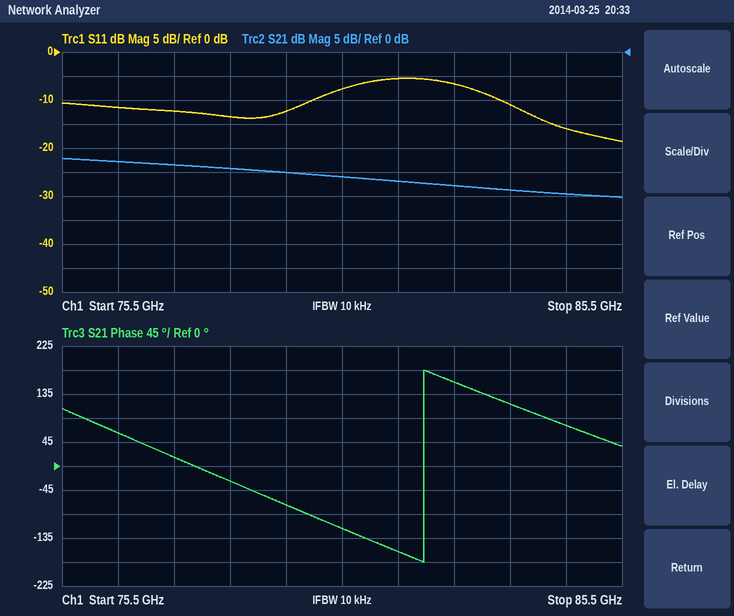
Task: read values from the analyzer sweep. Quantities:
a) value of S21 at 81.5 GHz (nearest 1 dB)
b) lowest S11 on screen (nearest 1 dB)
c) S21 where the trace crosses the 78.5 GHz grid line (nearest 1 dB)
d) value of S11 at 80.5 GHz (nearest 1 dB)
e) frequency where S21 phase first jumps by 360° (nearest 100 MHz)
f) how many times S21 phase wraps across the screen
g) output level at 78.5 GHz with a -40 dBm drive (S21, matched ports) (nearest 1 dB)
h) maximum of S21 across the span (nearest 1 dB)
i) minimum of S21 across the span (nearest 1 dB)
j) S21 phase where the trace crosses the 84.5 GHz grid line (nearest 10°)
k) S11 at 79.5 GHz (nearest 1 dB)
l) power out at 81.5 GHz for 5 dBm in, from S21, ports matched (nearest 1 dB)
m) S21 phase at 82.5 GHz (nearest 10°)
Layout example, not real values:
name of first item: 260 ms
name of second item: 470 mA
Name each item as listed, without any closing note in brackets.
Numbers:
value of S21 at 81.5 GHz: -27 dB
lowest S11 on screen: -19 dB
S21 where the trace crosses the 78.5 GHz grid line: -24 dB
value of S11 at 80.5 GHz: -8 dB
frequency where S21 phase first jumps by 360°: 82.0 GHz
how many times S21 phase wraps across the screen: 1
output level at 78.5 GHz with a -40 dBm drive (S21, matched ports): -64 dBm
maximum of S21 across the span: -22 dB
minimum of S21 across the span: -30 dB
S21 phase where the trace crosses the 84.5 GHz grid line: 80°
S11 at 79.5 GHz: -12 dB
power out at 81.5 GHz for 5 dBm in, from S21, ports matched: -22 dBm
S21 phase at 82.5 GHz: 160°
